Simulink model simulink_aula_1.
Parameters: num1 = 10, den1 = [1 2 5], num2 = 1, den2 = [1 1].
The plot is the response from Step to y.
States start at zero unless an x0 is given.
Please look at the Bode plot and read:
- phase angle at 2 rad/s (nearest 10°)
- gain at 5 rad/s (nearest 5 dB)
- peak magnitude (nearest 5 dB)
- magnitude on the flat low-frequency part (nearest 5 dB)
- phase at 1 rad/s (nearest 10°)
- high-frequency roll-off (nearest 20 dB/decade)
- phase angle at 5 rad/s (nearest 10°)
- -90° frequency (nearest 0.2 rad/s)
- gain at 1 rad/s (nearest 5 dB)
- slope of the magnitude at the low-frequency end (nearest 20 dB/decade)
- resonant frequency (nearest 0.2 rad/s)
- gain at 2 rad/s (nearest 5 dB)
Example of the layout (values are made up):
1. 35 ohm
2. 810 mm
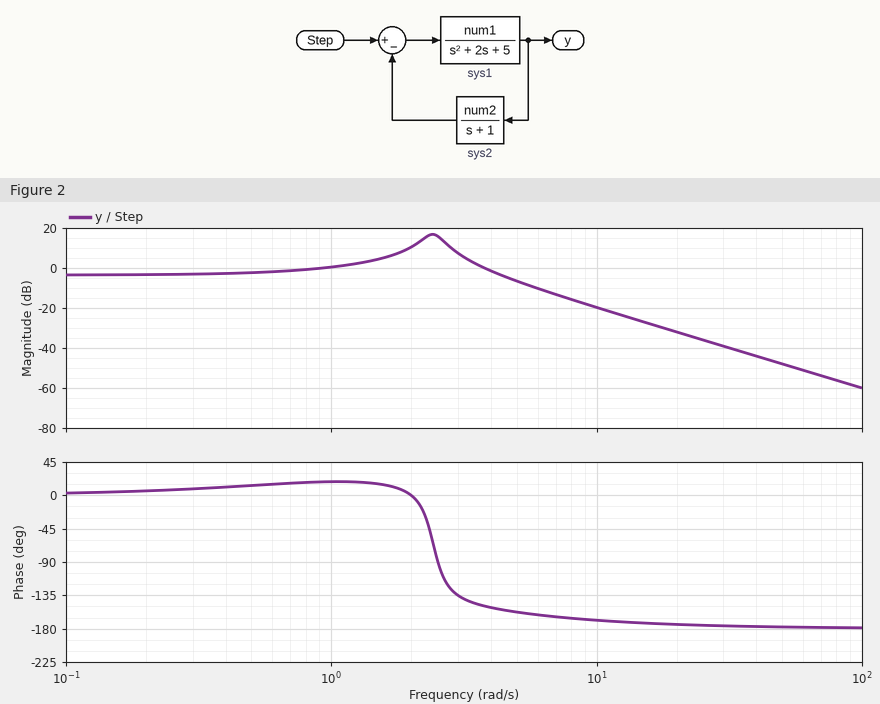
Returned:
1. 0°
2. -5 dB
3. 15 dB
4. -5 dB
5. 20°
6. -40 dB/decade
7. -160°
8. 2.6 rad/s
9. 0 dB
10. 0 dB/decade
11. 2.4 rad/s
12. 10 dB
